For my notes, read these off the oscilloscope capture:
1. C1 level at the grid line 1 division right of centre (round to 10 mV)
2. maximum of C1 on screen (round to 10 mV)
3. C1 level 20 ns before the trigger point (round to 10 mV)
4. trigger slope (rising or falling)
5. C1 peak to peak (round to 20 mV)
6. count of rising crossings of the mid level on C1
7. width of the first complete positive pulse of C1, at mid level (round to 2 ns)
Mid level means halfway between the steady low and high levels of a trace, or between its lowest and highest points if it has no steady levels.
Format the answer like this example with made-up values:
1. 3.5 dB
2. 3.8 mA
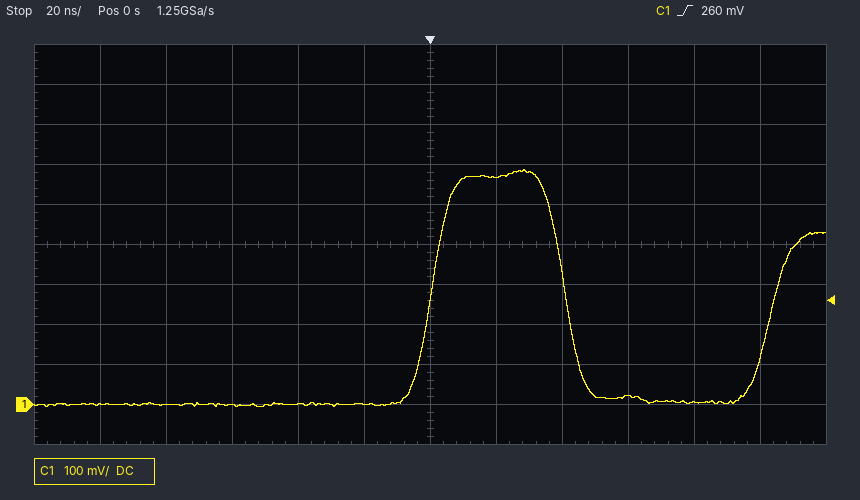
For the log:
1. 570 mV
2. 590 mV
3. 0 mV
4. rising
5. 600 mV
6. 2
7. 40 ns
